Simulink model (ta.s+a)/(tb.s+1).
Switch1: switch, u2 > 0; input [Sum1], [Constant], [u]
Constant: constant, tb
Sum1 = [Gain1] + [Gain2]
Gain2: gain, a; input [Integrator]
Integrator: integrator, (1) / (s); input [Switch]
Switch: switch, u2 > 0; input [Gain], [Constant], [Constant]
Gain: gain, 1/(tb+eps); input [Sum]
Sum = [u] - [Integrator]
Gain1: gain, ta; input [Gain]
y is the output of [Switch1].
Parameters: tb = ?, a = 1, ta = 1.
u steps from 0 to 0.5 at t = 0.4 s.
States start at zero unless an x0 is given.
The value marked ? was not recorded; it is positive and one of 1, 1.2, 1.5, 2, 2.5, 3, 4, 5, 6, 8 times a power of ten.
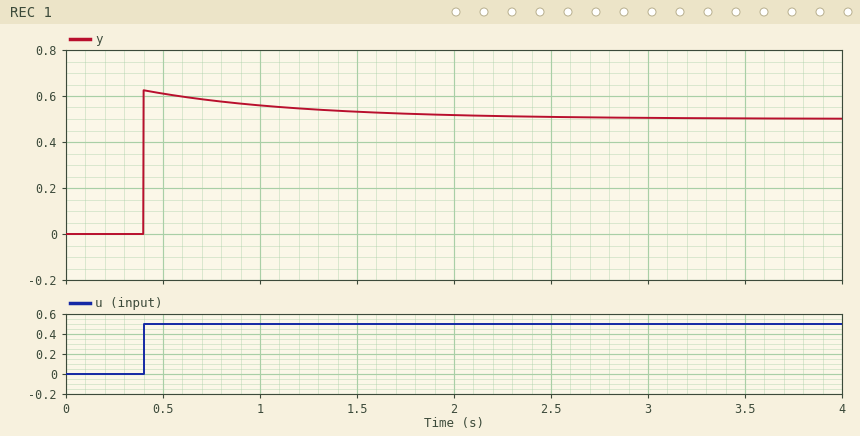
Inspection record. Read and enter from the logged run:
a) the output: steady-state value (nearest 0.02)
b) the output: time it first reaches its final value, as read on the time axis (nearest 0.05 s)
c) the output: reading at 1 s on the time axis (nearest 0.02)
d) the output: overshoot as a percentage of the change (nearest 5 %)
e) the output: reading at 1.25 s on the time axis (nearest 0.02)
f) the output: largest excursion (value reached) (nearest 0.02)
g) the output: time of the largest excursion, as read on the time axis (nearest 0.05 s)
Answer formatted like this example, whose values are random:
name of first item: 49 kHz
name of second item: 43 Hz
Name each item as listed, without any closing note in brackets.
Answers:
the output: steady-state value: 0.50
the output: time it first reaches its final value, as read on the time axis: 0.40 s
the output: reading at 1 s on the time axis: 0.56
the output: overshoot as a percentage of the change: 25 %
the output: reading at 1.25 s on the time axis: 0.54
the output: largest excursion (value reached): 0.62
the output: time of the largest excursion, as read on the time axis: 0.40 s
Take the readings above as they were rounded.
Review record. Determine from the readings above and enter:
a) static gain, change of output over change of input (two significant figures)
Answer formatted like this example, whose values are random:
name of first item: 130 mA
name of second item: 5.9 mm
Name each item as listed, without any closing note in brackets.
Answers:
static gain, change of output over change of input: 1.0
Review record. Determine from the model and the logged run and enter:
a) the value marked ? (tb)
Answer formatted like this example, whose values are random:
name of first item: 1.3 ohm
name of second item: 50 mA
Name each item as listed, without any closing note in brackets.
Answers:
the value marked ?: 0.8
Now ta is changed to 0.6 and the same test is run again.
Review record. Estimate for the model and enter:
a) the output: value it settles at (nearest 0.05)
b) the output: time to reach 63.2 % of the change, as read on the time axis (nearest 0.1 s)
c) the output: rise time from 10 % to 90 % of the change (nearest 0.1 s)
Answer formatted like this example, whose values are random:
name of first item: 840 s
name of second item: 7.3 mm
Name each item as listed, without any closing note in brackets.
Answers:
the output: value it settles at: 0.50
the output: time to reach 63.2 % of the change, as read on the time axis: 0.4 s
the output: rise time from 10 % to 90 % of the change: 0.7 s
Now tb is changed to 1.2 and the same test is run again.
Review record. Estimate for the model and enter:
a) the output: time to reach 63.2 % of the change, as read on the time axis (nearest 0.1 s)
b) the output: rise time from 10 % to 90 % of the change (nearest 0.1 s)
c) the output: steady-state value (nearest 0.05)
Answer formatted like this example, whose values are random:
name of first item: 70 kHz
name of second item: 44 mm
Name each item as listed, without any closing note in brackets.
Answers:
the output: time to reach 63.2 % of the change, as read on the time axis: 0.4 s
the output: rise time from 10 % to 90 % of the change: 0.6 s
the output: steady-state value: 0.50
